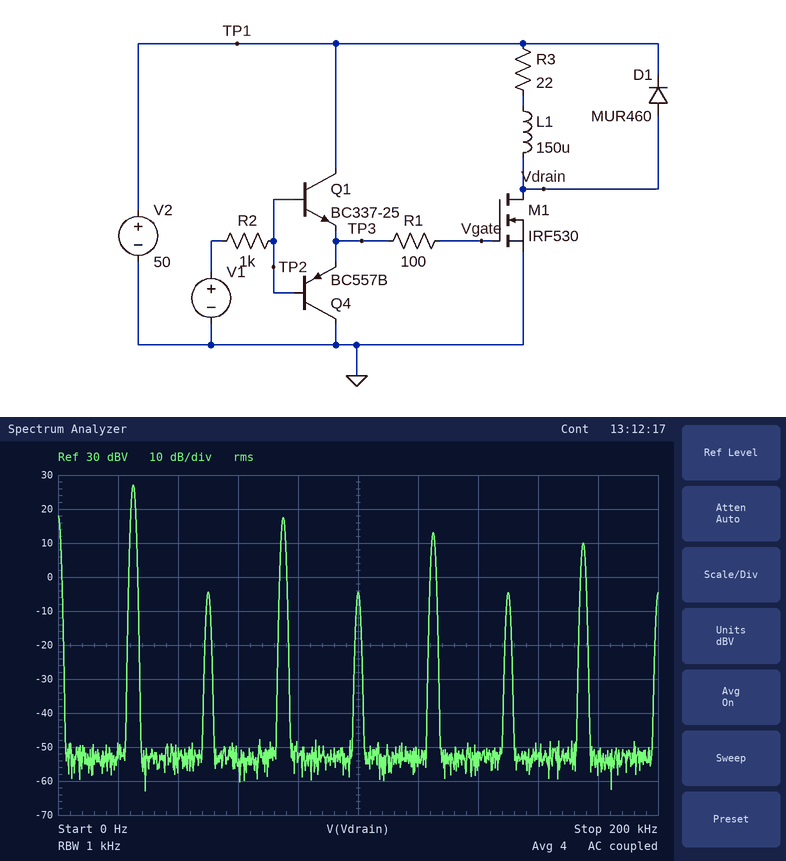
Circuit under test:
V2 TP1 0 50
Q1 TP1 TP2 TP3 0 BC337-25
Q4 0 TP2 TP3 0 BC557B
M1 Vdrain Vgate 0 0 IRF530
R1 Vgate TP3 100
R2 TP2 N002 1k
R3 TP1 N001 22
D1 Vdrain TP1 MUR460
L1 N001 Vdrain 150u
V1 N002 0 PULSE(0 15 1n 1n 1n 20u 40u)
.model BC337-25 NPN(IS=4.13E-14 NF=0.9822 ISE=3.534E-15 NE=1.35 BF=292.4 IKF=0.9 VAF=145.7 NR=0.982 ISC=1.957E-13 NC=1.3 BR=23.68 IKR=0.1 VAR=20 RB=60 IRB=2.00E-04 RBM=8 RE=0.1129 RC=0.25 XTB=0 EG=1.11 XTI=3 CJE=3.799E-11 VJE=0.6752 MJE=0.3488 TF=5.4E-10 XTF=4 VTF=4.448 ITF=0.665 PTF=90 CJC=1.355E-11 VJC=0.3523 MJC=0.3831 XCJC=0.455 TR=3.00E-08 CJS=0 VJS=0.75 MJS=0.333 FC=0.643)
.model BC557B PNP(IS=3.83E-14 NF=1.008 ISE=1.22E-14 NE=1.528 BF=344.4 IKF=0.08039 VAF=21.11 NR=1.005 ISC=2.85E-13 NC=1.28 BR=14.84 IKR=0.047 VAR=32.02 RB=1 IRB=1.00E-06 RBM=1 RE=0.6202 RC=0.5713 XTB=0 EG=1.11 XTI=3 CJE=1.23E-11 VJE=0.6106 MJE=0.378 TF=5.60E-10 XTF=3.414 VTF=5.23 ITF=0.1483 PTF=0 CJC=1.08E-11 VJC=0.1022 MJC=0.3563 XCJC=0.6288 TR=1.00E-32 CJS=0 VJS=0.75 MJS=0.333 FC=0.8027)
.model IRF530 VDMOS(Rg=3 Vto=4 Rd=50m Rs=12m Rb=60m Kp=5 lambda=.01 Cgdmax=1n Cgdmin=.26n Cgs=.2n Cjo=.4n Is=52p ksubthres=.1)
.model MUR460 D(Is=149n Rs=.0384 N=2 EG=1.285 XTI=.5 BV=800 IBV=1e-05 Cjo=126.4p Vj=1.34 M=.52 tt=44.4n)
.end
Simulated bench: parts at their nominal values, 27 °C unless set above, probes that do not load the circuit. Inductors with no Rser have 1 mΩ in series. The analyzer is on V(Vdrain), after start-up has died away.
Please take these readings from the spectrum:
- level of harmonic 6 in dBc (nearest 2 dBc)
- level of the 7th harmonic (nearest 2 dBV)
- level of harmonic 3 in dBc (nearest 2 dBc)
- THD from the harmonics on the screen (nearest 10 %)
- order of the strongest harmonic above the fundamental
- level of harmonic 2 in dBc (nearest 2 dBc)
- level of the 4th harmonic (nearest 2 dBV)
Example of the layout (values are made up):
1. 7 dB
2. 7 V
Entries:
1. -32 dBc
2. 10 dBV
3. -10 dBc
4. 40 %
5. 3
6. -32 dBc
7. -4 dBV
